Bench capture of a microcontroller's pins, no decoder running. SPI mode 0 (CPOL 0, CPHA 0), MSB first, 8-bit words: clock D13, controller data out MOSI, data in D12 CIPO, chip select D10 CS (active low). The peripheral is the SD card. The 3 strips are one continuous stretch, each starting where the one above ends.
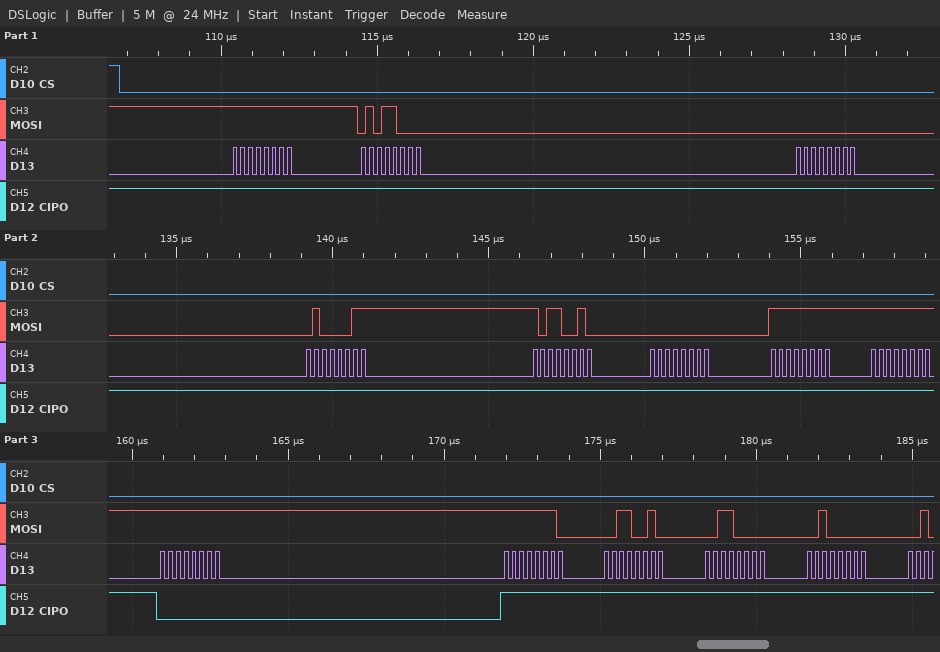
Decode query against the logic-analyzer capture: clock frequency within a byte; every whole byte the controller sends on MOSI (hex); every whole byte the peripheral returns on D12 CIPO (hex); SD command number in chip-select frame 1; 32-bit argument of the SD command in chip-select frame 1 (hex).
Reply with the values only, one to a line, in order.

4 MHz
FF 58 00 43 B2 00 FF FF FF FE 32 30 20
FF FF FF FF FF FF FF FF 00 FF FF FF FF
CMD24
0x0043B200
